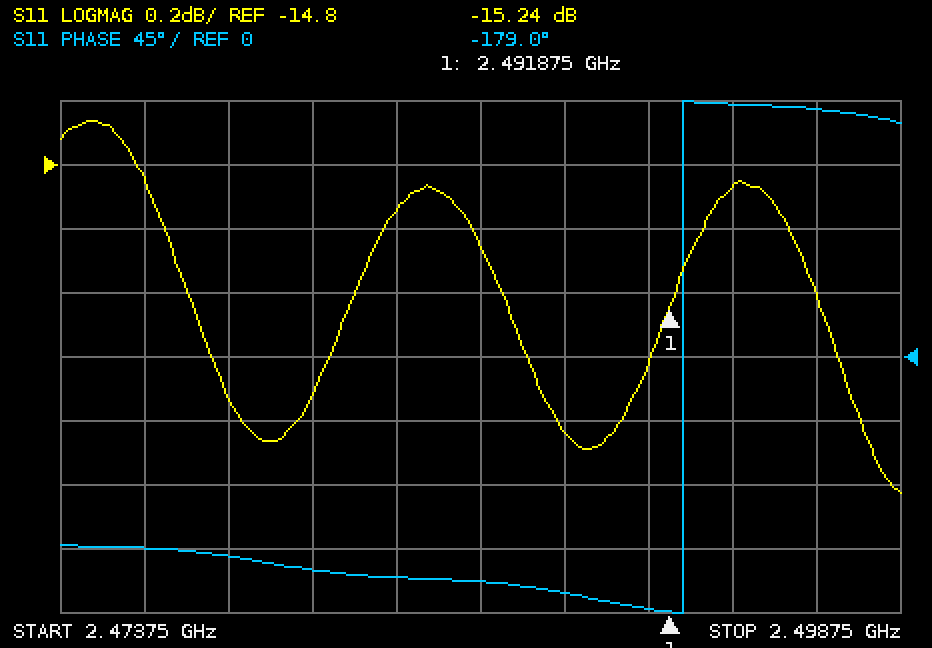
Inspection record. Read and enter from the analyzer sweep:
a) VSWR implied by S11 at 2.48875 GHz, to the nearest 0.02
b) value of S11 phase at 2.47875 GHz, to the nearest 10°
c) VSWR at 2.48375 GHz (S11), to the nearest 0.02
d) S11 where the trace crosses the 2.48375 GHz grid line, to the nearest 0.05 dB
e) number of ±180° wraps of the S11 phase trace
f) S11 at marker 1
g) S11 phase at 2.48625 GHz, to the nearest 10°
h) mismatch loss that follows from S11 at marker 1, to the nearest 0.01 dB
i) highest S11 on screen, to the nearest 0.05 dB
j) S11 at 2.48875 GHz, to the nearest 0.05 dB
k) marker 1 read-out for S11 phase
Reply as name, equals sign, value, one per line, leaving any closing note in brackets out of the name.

VSWR implied by S11 at 2.48875 GHz, to the nearest 0.02 = 1.40
value of S11 phase at 2.47875 GHz, to the nearest 10° = -140°
VSWR at 2.48375 GHz (S11), to the nearest 0.02 = 1.44
S11 where the trace crosses the 2.48375 GHz grid line, to the nearest 0.05 dB = -14.95 dB
number of ±180° wraps of the S11 phase trace = 1
S11 at marker 1 = -15.24 dB
S11 phase at 2.48625 GHz, to the nearest 10° = -160°
mismatch loss that follows from S11 at marker 1, to the nearest 0.01 dB = 0.13 dB
highest S11 on screen, to the nearest 0.05 dB = -14.65 dB
S11 at 2.48875 GHz, to the nearest 0.05 dB = -15.65 dB
marker 1 read-out for S11 phase = -179.0°
